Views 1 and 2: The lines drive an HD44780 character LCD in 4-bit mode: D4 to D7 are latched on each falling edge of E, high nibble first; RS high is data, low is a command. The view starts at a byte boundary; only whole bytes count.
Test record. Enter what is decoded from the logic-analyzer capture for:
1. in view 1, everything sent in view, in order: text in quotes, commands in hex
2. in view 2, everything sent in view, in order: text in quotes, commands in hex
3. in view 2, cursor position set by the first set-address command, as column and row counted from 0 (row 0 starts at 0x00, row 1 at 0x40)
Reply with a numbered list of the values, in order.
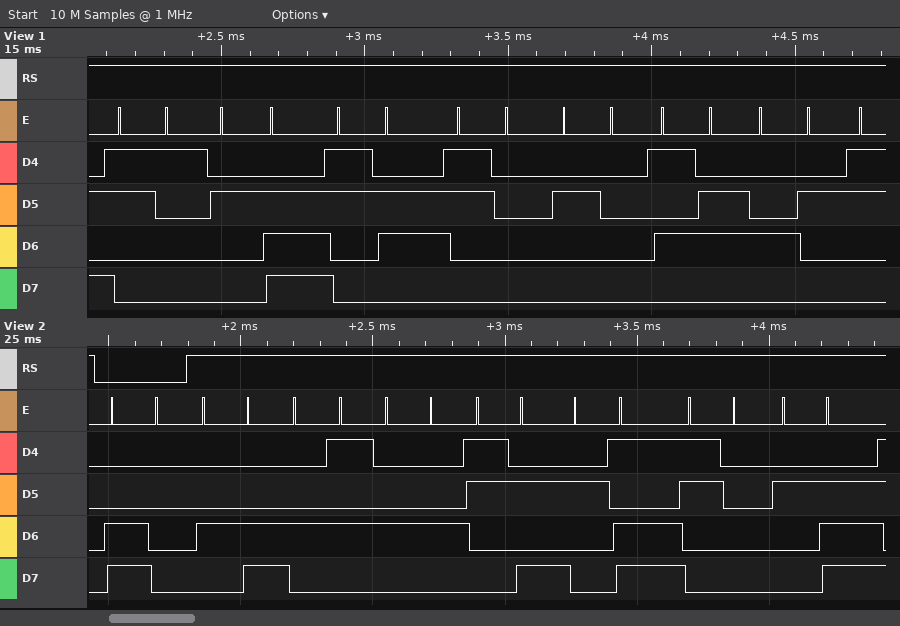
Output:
1. "1.60 VB"
2. 0xC0 "LED:-0."
3. column 0, row 1
